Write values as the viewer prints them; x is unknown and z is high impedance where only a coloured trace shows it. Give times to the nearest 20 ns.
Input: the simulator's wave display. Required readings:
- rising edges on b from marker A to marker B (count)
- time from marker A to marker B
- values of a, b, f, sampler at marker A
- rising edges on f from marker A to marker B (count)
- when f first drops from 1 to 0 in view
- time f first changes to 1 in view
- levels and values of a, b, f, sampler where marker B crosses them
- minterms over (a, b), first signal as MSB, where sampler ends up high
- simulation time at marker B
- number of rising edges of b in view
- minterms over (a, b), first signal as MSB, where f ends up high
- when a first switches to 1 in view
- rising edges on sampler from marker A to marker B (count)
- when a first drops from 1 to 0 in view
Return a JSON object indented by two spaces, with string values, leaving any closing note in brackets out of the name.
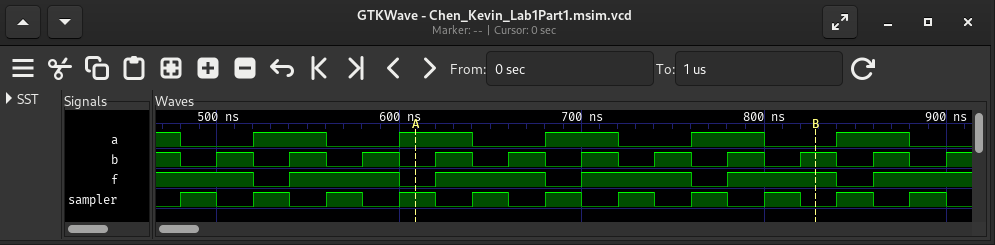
{
  "rising edges on b from marker A to marker B": "6",
  "time from marker A to marker B": "220 ns",
  "values of a, b, f, sampler at marker A": "a=1, b=0, f=0, sampler=1",
  "rising edges on f from marker A to marker B": "3",
  "when f first drops from 1 to 0 in view": "520 ns",
  "time f first changes to 1 in view": "540 ns",
  "levels and values of a, b, f, sampler where marker B crosses them": "a=0, b=1, f=1, sampler=0",
  "minterms over (a, b), first signal as MSB, where sampler ends up high": "0, 2",
  "simulation time at marker B": "820 ns",
  "number of rising edges of b in view": "11",
  "minterms over (a, b), first signal as MSB, where f ends up high": "0, 1, 3",
  "when a first switches to 1 in view": "520 ns",
  "rising edges on sampler from marker A to marker B": "5",
  "when a first drops from 1 to 0 in view": "480 ns"
}
